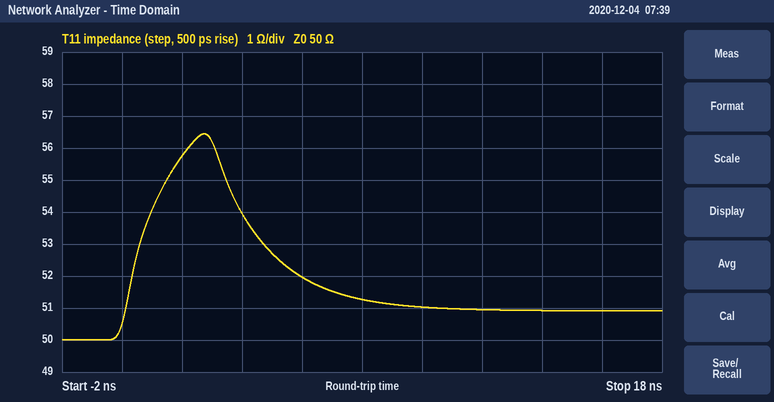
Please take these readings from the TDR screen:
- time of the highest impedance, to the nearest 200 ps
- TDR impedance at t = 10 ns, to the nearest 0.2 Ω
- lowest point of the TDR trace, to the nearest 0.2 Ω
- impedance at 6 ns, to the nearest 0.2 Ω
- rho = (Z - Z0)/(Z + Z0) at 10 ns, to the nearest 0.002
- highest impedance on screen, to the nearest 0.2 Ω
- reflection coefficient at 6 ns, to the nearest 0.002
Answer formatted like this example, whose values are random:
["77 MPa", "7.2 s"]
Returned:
["2.8 ns", "51.0 Ω", "50.0 Ω", "52.0 Ω", "+0.010", "56.4 Ω", "+0.020"]
